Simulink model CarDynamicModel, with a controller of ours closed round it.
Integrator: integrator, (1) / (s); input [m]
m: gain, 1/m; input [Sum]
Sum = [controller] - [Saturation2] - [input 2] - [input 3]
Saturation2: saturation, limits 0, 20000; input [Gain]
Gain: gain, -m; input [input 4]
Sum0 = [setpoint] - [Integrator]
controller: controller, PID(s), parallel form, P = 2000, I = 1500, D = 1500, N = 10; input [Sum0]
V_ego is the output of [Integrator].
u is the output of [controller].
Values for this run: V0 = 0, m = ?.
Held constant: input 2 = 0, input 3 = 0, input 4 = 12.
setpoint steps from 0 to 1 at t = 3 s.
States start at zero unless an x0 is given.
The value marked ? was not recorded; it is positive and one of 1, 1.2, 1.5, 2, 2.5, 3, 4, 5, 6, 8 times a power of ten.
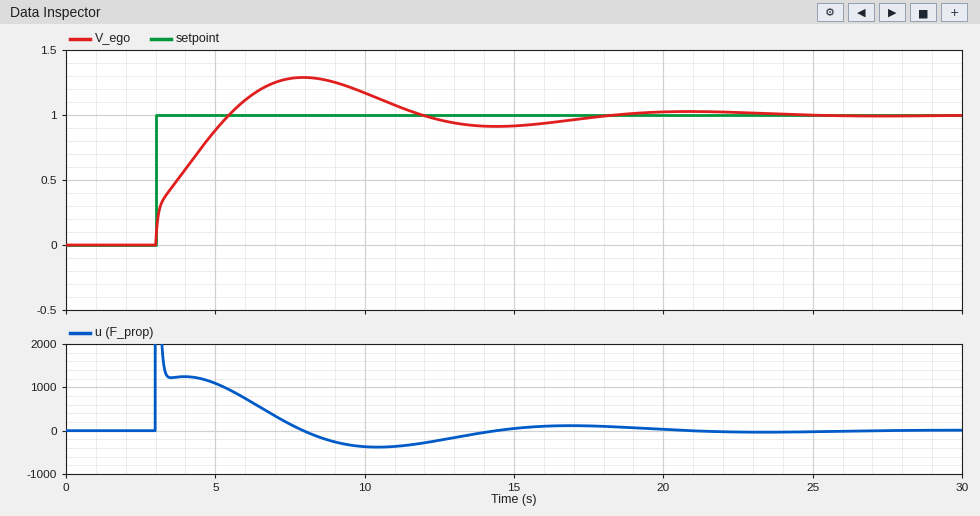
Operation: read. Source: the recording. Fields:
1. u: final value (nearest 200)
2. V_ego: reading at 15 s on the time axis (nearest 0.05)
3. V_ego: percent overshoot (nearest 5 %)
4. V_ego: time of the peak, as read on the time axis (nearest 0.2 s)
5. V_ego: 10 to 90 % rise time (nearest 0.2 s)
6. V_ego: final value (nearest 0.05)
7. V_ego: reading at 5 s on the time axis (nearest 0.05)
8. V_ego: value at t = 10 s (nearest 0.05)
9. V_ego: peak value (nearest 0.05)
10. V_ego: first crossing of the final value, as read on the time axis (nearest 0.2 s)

0
0.90
30 %
8.0 s
2.0 s
1.00
0.90
1.15
1.30
5.4 s
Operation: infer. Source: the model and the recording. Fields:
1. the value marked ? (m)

4000
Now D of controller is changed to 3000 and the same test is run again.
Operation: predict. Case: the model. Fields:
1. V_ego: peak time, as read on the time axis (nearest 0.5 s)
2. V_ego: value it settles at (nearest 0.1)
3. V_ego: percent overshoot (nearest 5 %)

8.5 s
1.0
25 %
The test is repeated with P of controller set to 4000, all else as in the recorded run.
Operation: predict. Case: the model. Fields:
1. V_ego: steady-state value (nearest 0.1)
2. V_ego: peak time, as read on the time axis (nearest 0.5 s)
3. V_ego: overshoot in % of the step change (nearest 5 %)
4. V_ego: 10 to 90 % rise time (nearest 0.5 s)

1.0
7.5 s
15 %
1.5 s
